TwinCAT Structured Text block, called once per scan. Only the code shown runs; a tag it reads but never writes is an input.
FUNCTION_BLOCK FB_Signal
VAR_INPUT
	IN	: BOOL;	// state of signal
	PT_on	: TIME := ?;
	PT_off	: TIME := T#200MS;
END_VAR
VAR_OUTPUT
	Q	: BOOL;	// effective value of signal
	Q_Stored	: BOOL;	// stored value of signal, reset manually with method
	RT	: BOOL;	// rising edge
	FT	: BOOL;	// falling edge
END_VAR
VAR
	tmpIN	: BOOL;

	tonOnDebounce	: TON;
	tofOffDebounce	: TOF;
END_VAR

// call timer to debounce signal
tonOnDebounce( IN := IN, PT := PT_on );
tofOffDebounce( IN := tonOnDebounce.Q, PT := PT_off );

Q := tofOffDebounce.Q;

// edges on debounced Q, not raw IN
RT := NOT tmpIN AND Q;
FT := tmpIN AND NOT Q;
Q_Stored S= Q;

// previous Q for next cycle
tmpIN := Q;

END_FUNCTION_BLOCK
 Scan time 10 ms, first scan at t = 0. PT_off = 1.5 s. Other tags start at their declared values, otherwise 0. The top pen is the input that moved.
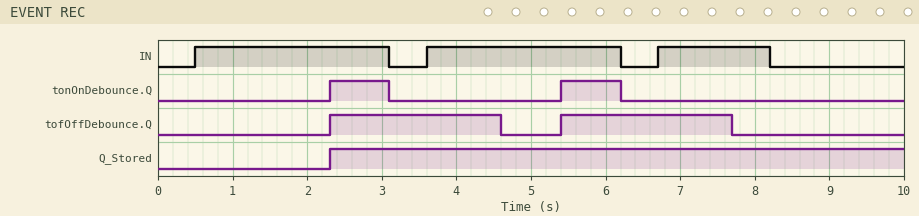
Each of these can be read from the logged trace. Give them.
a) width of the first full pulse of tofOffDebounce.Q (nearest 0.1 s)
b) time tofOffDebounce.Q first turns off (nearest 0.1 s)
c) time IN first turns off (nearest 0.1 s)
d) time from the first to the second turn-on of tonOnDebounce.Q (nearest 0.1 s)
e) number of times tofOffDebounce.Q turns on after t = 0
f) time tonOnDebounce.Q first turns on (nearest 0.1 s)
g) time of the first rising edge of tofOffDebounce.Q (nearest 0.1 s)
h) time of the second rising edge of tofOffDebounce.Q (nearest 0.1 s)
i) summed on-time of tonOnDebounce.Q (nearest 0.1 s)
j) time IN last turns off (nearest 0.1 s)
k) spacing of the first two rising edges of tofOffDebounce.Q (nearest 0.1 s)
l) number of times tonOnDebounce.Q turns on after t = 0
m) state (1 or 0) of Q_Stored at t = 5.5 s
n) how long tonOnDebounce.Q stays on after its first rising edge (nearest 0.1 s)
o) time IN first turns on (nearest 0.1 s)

2.3 s
4.6 s
3.1 s
3.1 s
2
2.3 s
2.3 s
5.4 s
1.6 s
8.2 s
3.1 s
2
1
0.8 s
0.5 s
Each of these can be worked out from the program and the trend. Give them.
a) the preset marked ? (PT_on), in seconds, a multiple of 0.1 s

1.8 s
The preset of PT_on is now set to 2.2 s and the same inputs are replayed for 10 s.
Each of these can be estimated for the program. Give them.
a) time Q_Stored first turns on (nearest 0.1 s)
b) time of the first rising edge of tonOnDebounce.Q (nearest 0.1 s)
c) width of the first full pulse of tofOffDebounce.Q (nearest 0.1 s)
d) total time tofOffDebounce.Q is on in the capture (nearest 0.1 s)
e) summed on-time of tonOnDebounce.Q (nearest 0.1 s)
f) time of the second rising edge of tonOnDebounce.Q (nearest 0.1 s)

2.7 s
2.7 s
1.9 s
3.8 s
0.8 s
5.8 s
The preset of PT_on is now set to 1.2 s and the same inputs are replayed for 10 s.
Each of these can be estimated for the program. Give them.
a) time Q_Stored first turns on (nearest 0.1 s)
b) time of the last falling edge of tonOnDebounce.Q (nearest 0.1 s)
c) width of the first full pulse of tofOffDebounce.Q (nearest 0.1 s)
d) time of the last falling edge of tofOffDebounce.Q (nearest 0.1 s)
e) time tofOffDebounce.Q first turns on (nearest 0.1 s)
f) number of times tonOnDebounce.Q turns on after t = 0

1.7 s
8.2 s
2.9 s
9.7 s
1.7 s
3
